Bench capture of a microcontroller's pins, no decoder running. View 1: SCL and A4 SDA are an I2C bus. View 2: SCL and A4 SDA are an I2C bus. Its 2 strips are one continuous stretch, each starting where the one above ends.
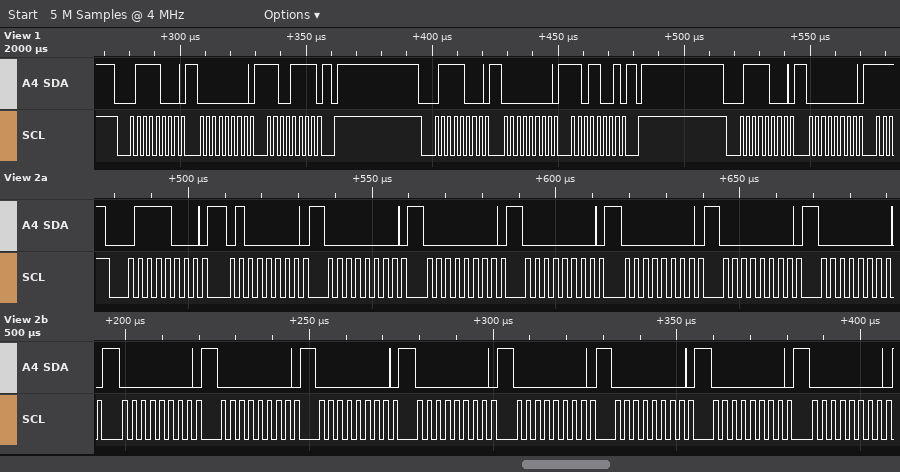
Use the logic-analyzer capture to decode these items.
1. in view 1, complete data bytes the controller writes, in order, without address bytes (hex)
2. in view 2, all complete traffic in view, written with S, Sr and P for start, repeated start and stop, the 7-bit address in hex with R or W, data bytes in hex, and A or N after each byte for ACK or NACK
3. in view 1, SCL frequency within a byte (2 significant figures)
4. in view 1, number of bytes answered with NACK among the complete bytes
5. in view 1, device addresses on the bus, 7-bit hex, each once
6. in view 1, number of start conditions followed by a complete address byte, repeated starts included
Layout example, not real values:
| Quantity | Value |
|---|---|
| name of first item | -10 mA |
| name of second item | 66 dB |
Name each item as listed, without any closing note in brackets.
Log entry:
| Quantity | Value |
|---|---|
| in view 1, complete data bytes the controller writes, in order, without address bytes | 00 CF 00 D9 00 |
| in view 2, all complete traffic in view, written with S, Sr and P for start, repeated start and stop, the 7-bit address in hex with R or W, data bytes in hex, and A or N after each byte for ACK or NACK | S 3CW A 40 A 00 A 00 A 00 A 00 A 00 A 00 A 00 A 00 A 00 A 00 A 00 A 00 A 00 A 00 A |
| in view 1, SCL frequency within a byte | 400 kHz |
| in view 1, number of bytes answered with NACK among the complete bytes | 0 |
| in view 1, device addresses on the bus, 7-bit hex, each once | 0x3C |
| in view 1, number of start conditions followed by a complete address byte, repeated starts included | 3 |
